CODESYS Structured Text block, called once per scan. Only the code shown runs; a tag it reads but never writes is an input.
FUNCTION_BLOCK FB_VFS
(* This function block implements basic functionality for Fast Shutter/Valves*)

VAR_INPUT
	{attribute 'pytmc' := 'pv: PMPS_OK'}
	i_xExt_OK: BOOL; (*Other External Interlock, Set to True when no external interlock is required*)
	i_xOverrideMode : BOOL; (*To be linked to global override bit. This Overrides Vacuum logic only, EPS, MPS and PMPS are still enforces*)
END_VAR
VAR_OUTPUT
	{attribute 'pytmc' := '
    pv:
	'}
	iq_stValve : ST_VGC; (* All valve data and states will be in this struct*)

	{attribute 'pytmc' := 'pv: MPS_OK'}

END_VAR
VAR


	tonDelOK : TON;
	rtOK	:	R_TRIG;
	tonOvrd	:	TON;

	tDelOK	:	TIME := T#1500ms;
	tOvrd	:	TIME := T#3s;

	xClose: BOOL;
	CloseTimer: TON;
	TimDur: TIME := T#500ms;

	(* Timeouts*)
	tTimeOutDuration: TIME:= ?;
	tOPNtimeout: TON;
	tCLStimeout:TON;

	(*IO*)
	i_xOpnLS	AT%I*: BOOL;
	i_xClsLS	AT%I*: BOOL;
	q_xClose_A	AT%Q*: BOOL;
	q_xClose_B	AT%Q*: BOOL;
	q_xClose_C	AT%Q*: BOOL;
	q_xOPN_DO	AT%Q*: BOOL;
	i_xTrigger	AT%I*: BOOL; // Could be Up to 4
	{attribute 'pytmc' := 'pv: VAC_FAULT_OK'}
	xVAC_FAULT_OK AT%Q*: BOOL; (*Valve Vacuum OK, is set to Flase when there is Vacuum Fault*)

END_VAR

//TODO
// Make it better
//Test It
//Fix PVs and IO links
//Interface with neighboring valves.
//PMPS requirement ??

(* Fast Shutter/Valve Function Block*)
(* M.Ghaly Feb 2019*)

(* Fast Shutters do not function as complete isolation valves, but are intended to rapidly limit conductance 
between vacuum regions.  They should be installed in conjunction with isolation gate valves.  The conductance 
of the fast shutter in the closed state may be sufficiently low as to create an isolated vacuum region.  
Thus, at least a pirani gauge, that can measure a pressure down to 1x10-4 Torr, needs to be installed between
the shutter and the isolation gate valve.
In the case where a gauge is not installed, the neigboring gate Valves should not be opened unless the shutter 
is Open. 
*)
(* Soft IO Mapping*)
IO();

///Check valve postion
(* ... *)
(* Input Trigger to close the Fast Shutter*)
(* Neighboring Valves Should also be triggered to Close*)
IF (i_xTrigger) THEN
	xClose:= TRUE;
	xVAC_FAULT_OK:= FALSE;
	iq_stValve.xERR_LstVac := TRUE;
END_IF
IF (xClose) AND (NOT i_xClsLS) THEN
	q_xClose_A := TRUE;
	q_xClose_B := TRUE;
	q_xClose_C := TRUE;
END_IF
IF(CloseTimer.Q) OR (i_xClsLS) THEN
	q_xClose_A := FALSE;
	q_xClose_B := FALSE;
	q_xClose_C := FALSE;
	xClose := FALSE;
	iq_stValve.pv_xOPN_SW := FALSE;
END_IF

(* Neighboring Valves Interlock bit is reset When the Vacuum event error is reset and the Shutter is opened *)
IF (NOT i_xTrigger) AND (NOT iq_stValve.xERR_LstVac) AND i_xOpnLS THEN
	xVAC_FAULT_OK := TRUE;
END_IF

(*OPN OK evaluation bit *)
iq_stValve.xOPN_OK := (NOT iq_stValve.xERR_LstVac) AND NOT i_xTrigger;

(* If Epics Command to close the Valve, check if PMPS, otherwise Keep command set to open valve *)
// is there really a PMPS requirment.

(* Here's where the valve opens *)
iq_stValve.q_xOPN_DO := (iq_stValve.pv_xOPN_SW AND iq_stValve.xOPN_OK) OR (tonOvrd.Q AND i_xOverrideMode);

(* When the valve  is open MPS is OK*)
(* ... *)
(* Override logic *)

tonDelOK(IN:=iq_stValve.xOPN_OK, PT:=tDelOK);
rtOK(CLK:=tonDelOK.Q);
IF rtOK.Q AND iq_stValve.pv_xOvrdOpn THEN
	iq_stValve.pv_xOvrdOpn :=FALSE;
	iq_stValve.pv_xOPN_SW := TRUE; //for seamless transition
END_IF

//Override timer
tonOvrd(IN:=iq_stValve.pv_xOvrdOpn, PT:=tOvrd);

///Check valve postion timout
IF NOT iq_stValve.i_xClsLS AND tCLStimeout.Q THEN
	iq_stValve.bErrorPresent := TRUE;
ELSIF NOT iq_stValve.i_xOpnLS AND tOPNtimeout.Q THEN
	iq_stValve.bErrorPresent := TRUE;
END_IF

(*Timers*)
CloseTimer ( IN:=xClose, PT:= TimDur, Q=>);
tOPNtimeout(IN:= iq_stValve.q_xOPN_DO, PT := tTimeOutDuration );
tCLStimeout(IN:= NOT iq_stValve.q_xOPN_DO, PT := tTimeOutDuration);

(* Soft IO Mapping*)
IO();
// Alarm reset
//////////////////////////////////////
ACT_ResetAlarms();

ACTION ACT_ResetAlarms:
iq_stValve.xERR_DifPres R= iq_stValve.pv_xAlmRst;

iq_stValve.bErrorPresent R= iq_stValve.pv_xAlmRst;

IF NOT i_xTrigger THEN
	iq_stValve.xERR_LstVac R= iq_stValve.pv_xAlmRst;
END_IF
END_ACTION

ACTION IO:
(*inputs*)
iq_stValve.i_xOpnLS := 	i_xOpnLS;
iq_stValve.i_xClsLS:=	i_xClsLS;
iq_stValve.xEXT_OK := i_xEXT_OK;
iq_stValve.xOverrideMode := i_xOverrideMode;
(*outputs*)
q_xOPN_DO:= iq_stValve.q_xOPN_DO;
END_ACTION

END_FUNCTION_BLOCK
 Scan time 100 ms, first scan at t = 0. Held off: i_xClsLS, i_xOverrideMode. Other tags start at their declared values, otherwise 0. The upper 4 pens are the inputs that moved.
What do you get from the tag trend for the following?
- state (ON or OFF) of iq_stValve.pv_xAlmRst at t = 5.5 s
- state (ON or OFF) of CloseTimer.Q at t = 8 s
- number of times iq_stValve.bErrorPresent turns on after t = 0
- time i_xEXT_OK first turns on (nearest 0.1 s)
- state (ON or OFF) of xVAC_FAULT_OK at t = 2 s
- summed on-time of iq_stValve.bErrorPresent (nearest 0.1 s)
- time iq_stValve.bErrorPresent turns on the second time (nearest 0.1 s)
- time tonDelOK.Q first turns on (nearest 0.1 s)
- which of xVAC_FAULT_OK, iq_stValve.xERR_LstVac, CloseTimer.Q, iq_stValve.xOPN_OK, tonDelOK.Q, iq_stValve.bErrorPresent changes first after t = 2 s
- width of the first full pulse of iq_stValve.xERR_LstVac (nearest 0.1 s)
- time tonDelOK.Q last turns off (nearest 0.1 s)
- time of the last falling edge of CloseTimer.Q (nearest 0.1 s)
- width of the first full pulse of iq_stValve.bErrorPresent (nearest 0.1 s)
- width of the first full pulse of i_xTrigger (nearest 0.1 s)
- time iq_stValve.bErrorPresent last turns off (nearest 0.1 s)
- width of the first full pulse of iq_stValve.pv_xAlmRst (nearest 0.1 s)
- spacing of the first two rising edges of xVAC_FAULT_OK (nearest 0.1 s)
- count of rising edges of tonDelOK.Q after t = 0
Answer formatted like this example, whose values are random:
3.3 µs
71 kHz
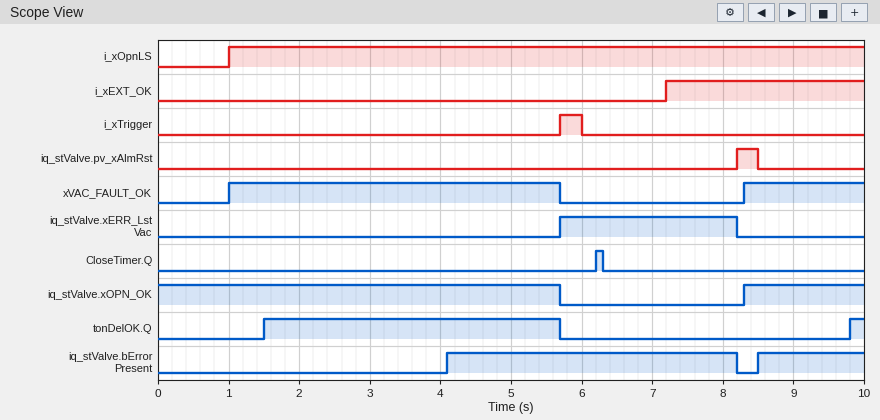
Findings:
OFF
OFF
2
7.2 s
ON
5.6 s
8.5 s
1.5 s
iq_stValve.bErrorPresent
2.5 s
5.7 s
6.3 s
4.1 s
0.3 s
8.2 s
0.3 s
7.3 s
2
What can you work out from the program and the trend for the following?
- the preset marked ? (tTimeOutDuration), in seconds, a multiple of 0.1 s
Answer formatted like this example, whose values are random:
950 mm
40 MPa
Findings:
4.0 s
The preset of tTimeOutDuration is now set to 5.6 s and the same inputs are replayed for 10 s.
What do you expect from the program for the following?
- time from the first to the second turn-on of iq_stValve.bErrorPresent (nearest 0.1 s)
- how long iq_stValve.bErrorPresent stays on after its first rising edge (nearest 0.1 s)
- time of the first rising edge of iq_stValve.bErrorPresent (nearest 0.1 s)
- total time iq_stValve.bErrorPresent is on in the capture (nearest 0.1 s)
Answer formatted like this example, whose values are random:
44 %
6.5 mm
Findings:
2.8 s
2.5 s
5.7 s
4.0 s
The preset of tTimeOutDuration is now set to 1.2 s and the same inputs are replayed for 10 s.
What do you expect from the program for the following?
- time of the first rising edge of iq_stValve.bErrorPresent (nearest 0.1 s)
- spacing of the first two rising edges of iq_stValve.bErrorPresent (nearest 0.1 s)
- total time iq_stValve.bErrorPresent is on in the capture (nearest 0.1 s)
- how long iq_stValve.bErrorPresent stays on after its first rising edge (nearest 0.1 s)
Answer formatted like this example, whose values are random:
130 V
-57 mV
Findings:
1.3 s
7.2 s
8.4 s
6.9 s
